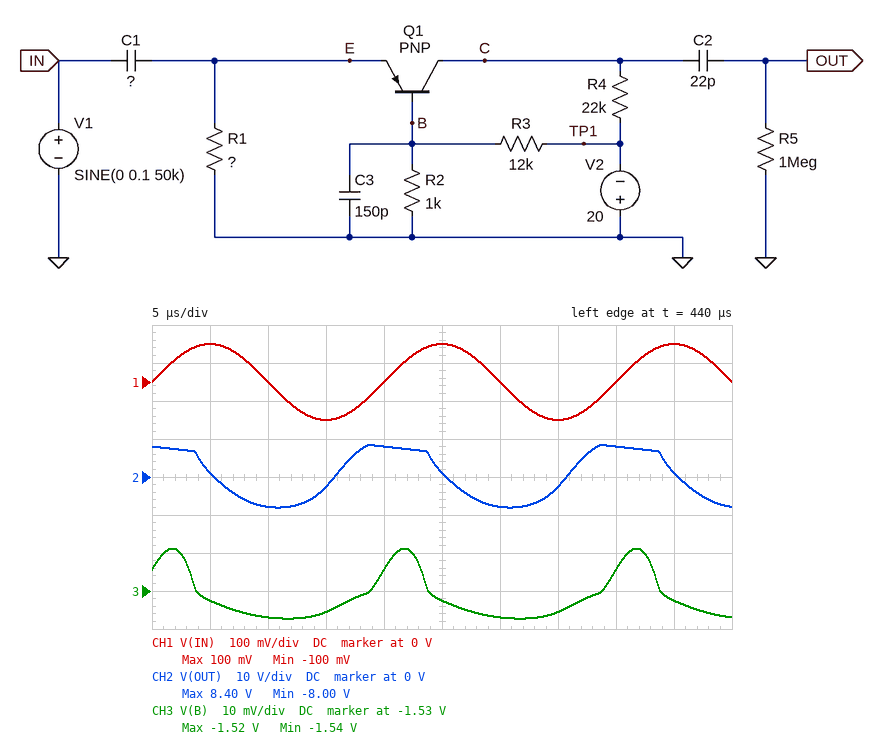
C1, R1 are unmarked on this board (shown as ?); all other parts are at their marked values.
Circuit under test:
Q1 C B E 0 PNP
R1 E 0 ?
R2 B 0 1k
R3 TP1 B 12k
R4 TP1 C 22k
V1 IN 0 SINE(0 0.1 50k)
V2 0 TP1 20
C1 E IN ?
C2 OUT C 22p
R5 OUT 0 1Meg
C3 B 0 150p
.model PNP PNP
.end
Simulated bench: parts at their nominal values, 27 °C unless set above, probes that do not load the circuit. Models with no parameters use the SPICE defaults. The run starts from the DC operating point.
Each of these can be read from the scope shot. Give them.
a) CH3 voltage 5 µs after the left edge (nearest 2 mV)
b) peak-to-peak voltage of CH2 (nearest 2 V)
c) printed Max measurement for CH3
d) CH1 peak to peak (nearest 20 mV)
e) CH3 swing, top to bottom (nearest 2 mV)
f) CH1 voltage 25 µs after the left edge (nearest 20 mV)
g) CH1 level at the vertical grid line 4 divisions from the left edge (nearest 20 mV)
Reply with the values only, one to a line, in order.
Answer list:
-1.532 V
16 V
-1.52 V
200 mV
18 mV
100 mV
0 V
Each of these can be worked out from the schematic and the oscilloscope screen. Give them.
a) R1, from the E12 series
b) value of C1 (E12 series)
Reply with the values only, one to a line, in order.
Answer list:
1.5 kΩ
15 nF
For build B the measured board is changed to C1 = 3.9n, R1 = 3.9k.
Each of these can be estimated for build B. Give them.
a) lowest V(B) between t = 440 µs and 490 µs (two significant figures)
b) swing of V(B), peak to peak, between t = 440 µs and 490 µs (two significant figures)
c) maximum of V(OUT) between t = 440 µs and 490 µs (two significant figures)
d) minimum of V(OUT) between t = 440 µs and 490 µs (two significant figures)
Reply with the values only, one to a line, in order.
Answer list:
-1.5 V
2.1 mV
2.5 V
-2.4 V
